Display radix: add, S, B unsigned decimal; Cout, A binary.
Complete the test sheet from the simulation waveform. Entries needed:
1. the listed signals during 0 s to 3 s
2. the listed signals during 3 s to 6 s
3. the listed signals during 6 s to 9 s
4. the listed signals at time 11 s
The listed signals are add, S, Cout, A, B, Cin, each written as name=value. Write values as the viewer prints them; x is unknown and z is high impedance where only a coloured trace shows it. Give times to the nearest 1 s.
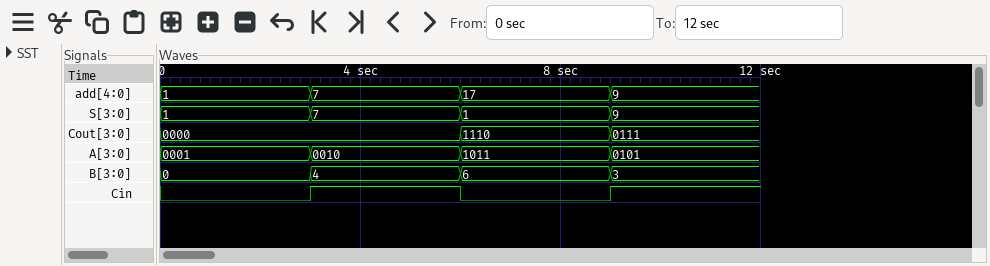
add=1, S=1, Cout=0000, A=0001, B=0, Cin=0
add=7, S=7, Cout=0000, A=0010, B=4, Cin=1
add=17, S=1, Cout=1110, A=1011, B=6, Cin=0
add=9, S=9, Cout=0111, A=0101, B=3, Cin=1
